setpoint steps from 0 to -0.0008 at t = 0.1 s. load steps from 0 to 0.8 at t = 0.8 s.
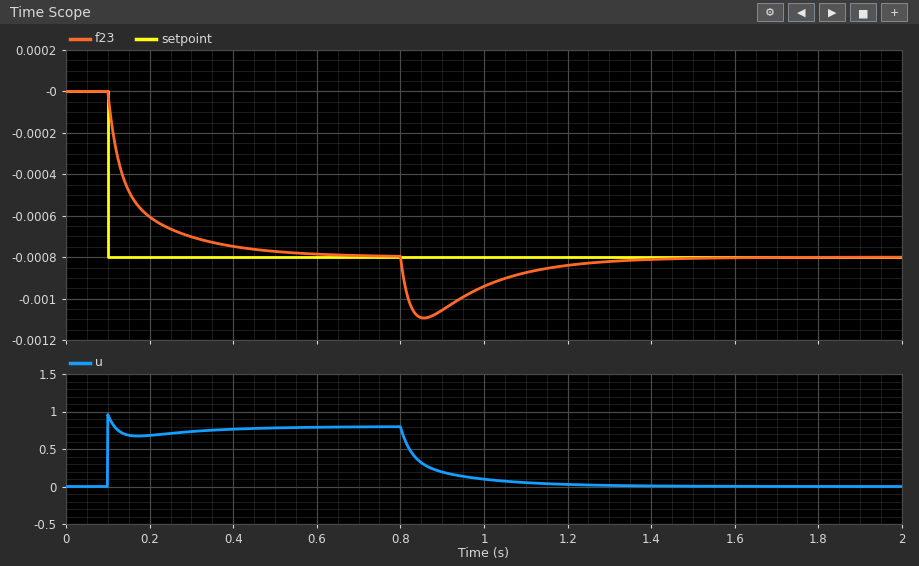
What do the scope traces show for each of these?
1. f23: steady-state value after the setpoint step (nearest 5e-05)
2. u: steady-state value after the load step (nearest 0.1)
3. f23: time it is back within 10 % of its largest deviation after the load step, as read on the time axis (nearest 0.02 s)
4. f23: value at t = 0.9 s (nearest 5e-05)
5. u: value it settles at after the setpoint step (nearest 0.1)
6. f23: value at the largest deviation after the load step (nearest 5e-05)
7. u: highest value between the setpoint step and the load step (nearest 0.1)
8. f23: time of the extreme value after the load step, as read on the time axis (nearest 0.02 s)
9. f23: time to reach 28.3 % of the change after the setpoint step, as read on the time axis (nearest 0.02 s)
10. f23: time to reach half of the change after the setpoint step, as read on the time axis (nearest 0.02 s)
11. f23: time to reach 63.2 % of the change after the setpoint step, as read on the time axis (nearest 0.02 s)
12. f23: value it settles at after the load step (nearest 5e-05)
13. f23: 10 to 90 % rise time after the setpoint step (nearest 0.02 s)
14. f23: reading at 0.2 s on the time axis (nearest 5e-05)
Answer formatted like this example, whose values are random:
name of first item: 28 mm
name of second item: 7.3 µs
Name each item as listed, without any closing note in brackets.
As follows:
f23: steady-state value after the setpoint step: -0.00080
u: steady-state value after the load step: 0.0
f23: time it is back within 10 % of its largest deviation after the load step, as read on the time axis: 1.24 s
f23: value at t = 0.9 s: -0.00105
u: value it settles at after the setpoint step: 0.8
f23: value at the largest deviation after the load step: -0.00110
u: highest value between the setpoint step and the load step: 1.0
f23: time of the extreme value after the load step, as read on the time axis: 0.86 s
f23: time to reach 28.3 % of the change after the setpoint step, as read on the time axis: 0.12 s
f23: time to reach half of the change after the setpoint step, as read on the time axis: 0.14 s
f23: time to reach 63.2 % of the change after the setpoint step, as read on the time axis: 0.16 s
f23: value it settles at after the load step: -0.00080
f23: 10 to 90 % rise time after the setpoint step: 0.22 s
f23: reading at 0.2 s on the time axis: -0.00060
